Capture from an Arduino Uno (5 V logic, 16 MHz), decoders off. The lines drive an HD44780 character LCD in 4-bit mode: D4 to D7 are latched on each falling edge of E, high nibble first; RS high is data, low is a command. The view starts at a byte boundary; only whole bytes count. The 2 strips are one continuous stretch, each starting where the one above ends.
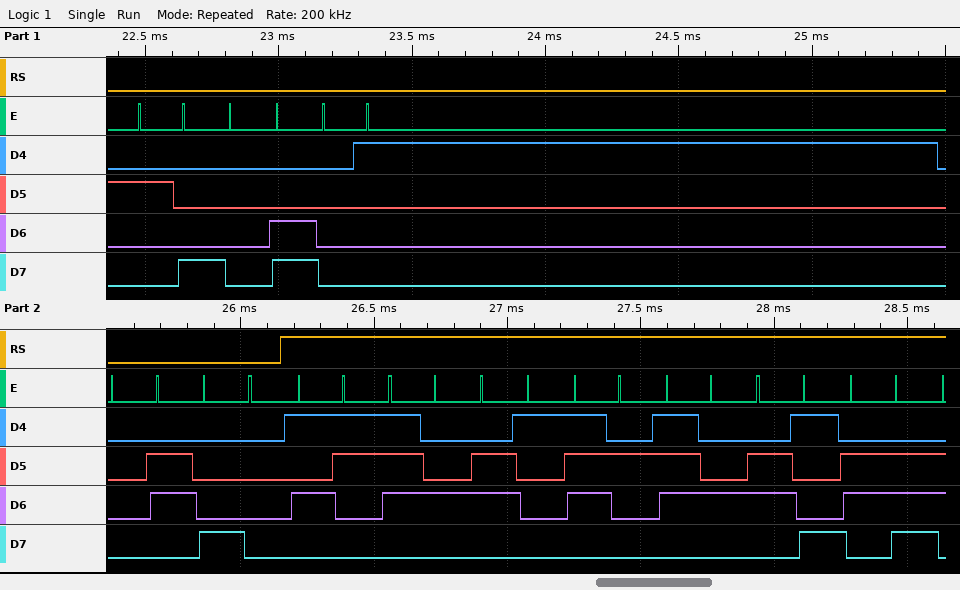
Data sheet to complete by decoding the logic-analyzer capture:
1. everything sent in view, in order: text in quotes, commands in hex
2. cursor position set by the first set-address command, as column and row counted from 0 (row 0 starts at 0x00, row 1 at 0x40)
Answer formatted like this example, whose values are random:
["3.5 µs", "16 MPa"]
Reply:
["0x28 0x0C 0x01 0x06 0x80 \"Startin\"", "column 0, row 0"]
